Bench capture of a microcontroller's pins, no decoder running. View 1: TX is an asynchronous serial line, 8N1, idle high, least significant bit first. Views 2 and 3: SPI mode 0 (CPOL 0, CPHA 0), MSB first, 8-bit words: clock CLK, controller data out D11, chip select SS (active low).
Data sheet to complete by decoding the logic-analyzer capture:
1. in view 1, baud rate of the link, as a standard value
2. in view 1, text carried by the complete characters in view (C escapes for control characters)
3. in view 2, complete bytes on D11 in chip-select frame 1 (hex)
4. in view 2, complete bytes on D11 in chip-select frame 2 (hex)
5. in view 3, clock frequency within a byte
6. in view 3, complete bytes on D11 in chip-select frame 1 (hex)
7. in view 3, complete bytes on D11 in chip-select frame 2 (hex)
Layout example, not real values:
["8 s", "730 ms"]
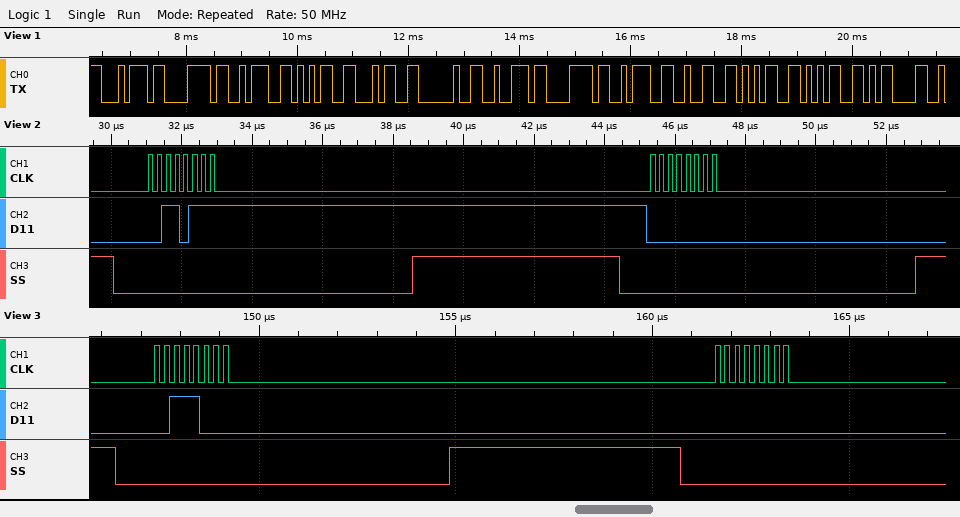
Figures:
["9600 baud", "\"tx:54 rx:255\\r\"", "37", "00", "4 MHz", "38", "00"]
